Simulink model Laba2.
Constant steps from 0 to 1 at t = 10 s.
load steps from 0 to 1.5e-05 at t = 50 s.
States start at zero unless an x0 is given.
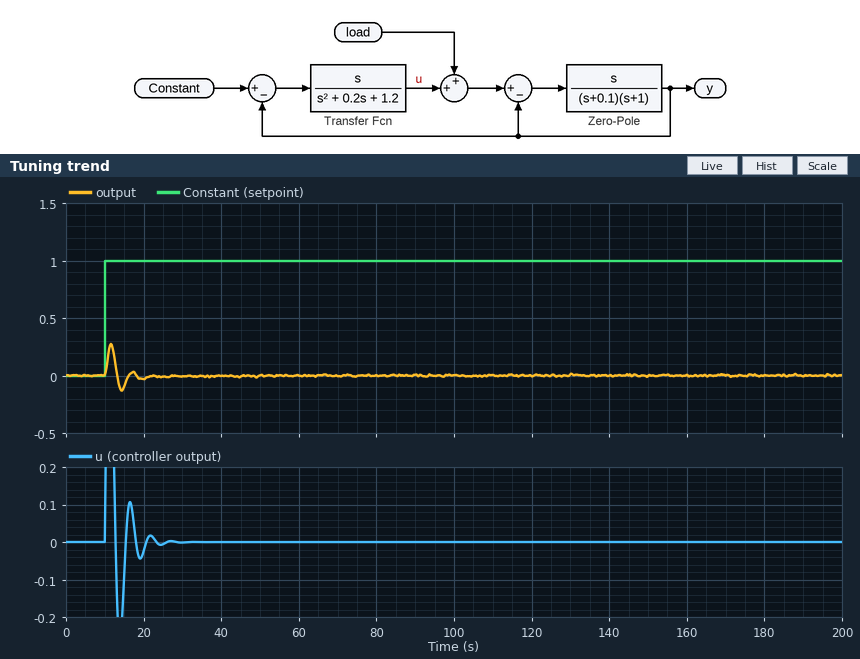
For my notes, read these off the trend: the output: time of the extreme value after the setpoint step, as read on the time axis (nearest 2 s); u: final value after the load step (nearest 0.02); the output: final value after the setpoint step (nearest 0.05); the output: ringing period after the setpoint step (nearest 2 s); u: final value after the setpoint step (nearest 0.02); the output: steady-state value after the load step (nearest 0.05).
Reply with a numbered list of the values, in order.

1. 12 s
2. 0.00
3. 0.00
4. 6 s
5. 0.00
6. 0.00
